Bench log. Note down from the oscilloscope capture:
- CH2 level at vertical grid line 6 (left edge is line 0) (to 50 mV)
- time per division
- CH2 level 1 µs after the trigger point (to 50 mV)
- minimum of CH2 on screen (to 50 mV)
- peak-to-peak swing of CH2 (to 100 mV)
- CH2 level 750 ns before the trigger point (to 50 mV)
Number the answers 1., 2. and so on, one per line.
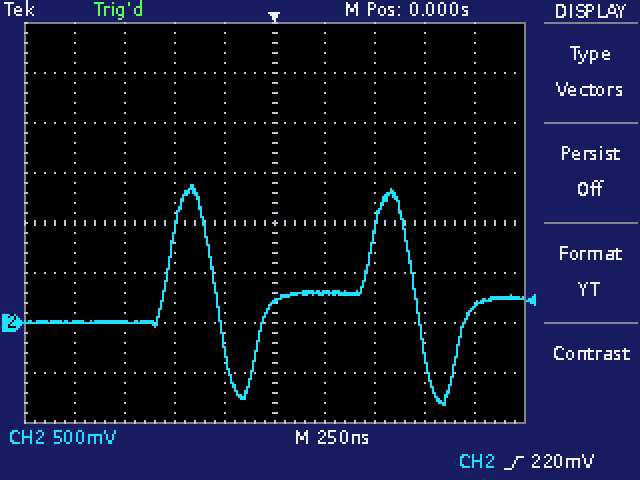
1. 300 mV
2. 250 ns
3. 150 mV
4. -800 mV
5. 2.20 V
6. 0 mV
